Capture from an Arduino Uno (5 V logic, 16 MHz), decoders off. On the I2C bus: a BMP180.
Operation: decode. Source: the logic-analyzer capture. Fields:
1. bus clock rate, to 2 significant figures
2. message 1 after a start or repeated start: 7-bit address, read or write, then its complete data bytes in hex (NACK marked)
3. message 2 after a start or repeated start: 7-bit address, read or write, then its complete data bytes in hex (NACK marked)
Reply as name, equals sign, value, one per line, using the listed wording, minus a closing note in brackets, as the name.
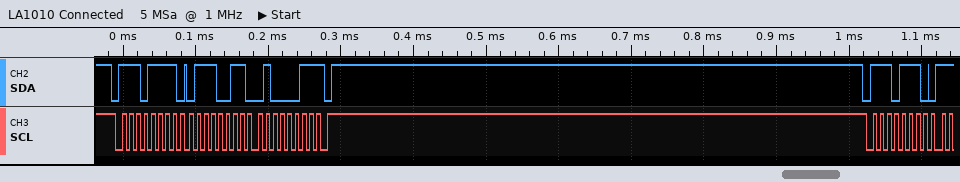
bus clock rate, to 2 significant figures = 100 kHz
message 1 after a start or repeated start: 7-bit address, read or write, then its complete data bytes in hex = 0x77 read: 73 43 NACK
message 2 after a start or repeated start: 7-bit address, read or write, then its complete data bytes in hex = 0x77 write
